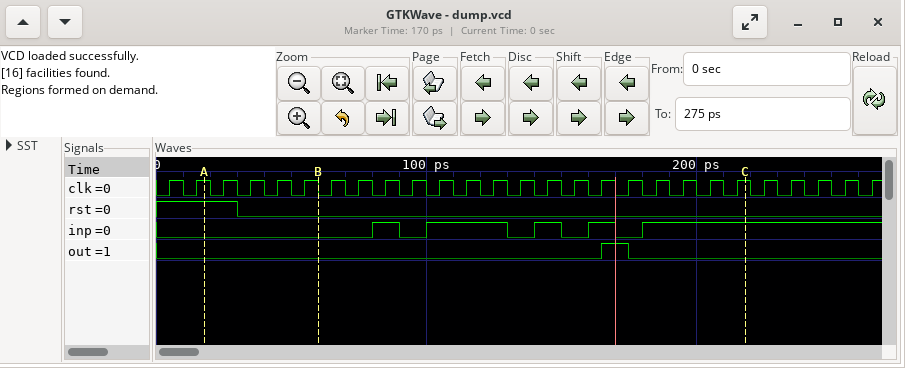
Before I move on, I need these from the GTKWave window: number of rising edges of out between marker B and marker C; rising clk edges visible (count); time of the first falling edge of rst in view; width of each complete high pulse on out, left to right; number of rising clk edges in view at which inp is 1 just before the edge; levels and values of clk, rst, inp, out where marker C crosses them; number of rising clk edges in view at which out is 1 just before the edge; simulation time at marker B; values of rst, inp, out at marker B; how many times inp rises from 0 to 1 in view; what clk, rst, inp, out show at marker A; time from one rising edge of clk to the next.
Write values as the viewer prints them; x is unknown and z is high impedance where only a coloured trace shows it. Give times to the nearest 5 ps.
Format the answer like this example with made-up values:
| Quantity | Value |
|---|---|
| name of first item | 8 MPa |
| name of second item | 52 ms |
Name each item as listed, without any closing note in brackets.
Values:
| Quantity | Value |
|---|---|
| number of rising edges of out between marker B and marker C | 1 |
| rising clk edges visible | 27 |
| time of the first falling edge of rst in view | 30 ps |
| width of each complete high pulse on out, left to right | 10 ps |
| number of rising clk edges in view at which inp is 1 just before the edge | 15 |
| levels and values of clk, rst, inp, out where marker C crosses them | clk=1, rst=0, inp=1, out=0 |
| number of rising clk edges in view at which out is 1 just before the edge | 1 |
| simulation time at marker B | 60 ps |
| values of rst, inp, out at marker B | rst=0, inp=0, out=0 |
| how many times inp rises from 0 to 1 in view | 5 |
| what clk, rst, inp, out show at marker A | clk=1, rst=1, inp=0, out=0 |
| time from one rising edge of clk to the next | 10 ps |
